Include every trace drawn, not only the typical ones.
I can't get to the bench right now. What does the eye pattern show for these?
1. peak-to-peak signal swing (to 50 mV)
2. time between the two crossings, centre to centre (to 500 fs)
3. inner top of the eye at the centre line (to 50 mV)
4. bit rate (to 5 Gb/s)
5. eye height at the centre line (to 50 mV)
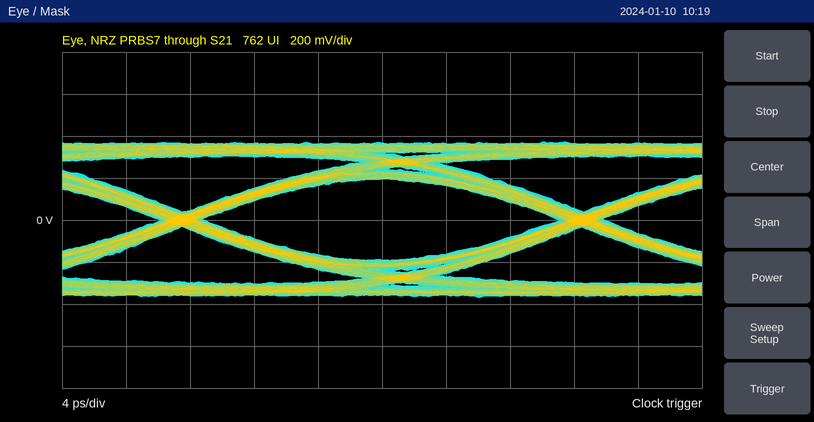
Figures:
750 mV
25.0 ps
200 mV
40 Gb/s
400 mV
